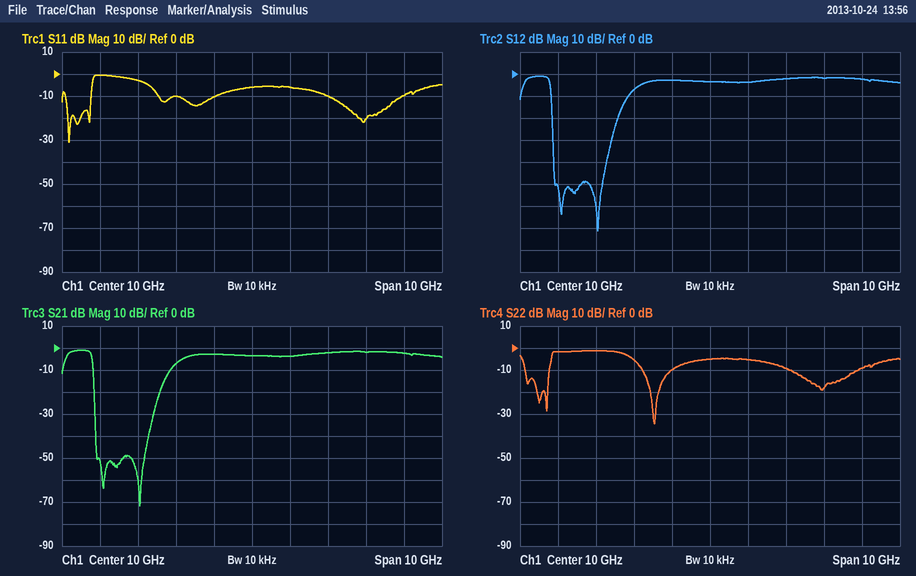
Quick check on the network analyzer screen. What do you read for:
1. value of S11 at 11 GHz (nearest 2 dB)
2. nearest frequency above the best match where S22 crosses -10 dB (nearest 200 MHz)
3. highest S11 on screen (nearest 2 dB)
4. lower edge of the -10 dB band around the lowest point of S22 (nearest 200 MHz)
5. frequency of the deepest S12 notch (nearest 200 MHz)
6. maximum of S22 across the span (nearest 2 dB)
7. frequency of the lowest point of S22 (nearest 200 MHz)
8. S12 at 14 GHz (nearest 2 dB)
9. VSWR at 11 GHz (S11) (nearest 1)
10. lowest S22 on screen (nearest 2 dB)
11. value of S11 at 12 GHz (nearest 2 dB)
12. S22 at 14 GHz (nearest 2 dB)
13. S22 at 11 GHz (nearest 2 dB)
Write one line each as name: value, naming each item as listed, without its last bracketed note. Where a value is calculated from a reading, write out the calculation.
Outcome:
value of S11 at 11 GHz: -6 dB
nearest frequency above the best match where S22 crosses -10 dB: 9.0 GHz
highest S11 on screen: 0 dB
lower edge of the -10 dB band around the lowest point of S22: 8.2 GHz
frequency of the deepest S12 notch: 7.0 GHz
maximum of S22 across the span: -2 dB
frequency of the lowest point of S22: 8.6 GHz
S12 at 14 GHz: -2 dB
VSWR at 11 GHz (S11): |Γ| = 10^(-6/20) = 0.5012; VSWR = (1 + 0.5012)/(1 − 0.5012) ≈ 3
lowest S22 on screen: -34 dB
value of S11 at 12 GHz: -10 dB
S22 at 14 GHz: -10 dB
S22 at 11 GHz: -6 dB
